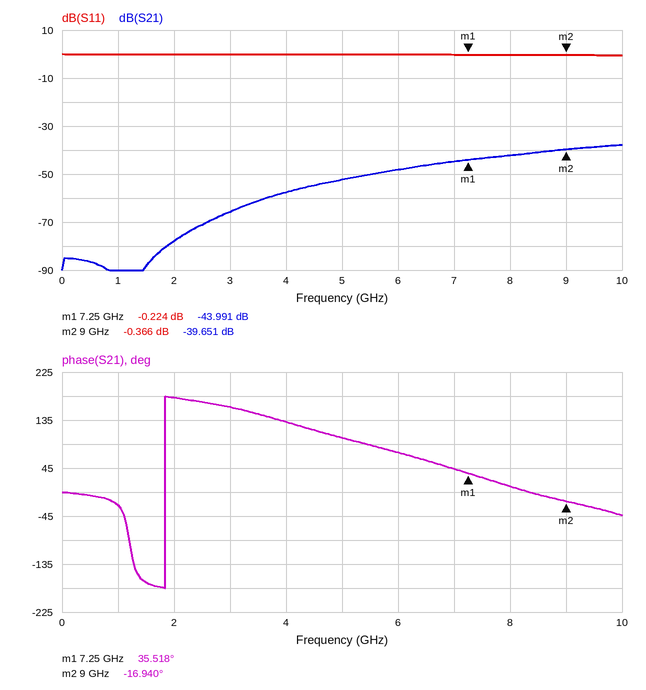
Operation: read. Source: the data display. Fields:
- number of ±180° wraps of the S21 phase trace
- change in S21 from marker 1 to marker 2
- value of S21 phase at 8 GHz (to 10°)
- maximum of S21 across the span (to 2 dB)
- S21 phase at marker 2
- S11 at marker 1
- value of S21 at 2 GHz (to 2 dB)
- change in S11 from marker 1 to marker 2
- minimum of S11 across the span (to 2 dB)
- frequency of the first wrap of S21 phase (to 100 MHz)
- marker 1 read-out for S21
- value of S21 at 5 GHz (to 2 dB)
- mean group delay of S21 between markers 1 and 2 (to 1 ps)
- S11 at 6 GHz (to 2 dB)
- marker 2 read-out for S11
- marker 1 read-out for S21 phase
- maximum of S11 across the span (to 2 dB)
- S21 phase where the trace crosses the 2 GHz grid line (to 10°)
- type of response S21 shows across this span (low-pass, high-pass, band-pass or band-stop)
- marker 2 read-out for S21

1
4.340 dB
10°
-38 dB
-16.940°
-0.224 dB
-78 dB
-0.142 dB
0 dB
1.8 GHz
-43.991 dB
-52 dB
83 ps
0 dB
-0.366 dB
35.518°
0 dB
180°
high-pass
-39.651 dB
